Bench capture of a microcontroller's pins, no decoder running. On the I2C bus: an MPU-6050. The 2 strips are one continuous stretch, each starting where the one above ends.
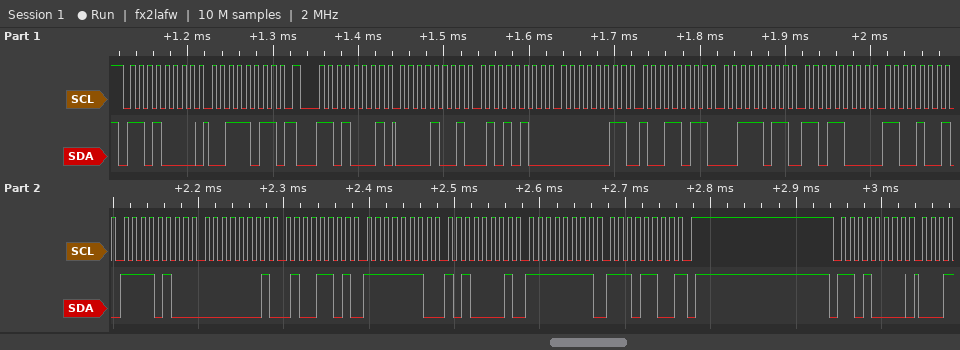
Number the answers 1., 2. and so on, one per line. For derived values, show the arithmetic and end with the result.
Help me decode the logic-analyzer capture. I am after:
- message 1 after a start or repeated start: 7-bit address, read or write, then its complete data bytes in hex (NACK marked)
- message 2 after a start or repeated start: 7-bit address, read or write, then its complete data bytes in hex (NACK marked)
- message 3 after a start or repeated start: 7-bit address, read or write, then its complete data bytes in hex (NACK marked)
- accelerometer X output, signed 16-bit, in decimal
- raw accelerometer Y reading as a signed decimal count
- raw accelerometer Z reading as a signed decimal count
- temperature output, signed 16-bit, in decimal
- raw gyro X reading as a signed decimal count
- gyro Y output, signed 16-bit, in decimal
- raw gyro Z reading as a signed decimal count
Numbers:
1. 0x68 write: 3B
2. 0x68 read: 09 54 03 9B 3B D8 C9 F4 01 4D FE A1 FF EC NACK
3. 0x68 write
4. 0x0954 = 2388
5. 0x039B = 923
6. 0x3BD8 = 15320
7. 0xC9F4 = -13836
8. 0x014D = 333
9. 0xFEA1 = -351
10. 0xFFEC = -20
